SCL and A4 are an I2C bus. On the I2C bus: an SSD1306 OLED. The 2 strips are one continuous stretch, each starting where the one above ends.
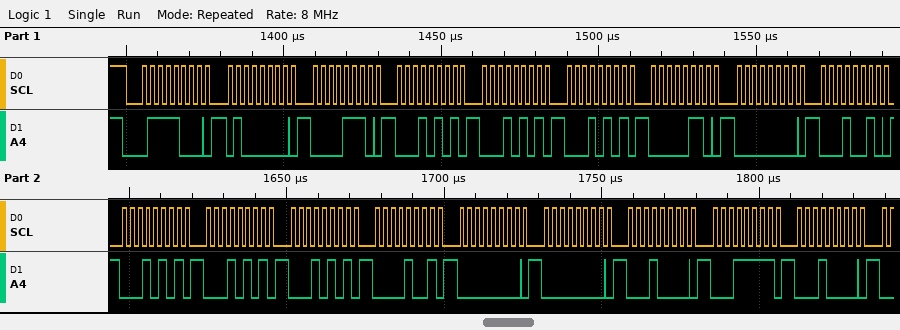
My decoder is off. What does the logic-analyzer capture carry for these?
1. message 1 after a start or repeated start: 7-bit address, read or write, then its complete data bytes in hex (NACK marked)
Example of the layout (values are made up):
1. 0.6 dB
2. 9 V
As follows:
1. 0x3C write: 40 0E 15 15 15 06 00 12 15 15 15 09 00 00 10 1F 10
